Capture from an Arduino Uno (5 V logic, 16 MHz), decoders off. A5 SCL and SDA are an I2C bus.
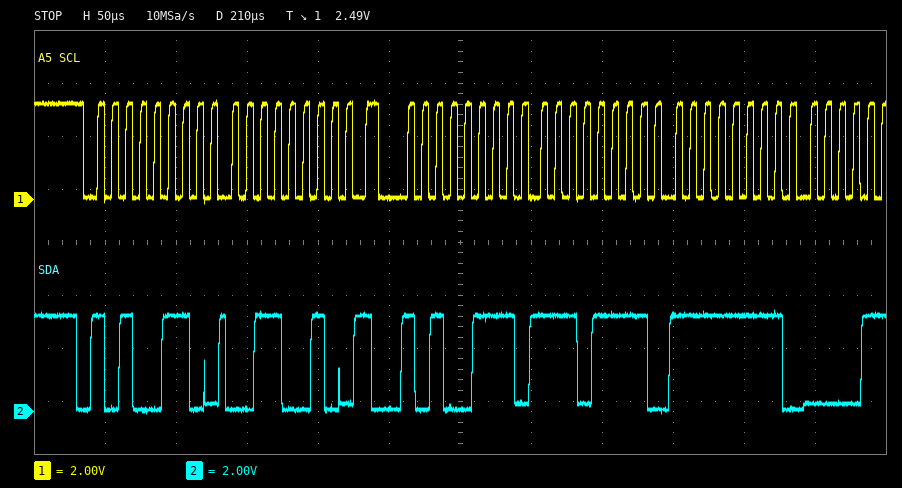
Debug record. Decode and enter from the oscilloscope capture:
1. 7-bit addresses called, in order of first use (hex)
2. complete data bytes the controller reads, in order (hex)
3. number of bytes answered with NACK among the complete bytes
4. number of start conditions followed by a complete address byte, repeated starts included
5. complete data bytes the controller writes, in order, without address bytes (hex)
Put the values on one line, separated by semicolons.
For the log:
0x53; EF FF; 0; 2; 32
